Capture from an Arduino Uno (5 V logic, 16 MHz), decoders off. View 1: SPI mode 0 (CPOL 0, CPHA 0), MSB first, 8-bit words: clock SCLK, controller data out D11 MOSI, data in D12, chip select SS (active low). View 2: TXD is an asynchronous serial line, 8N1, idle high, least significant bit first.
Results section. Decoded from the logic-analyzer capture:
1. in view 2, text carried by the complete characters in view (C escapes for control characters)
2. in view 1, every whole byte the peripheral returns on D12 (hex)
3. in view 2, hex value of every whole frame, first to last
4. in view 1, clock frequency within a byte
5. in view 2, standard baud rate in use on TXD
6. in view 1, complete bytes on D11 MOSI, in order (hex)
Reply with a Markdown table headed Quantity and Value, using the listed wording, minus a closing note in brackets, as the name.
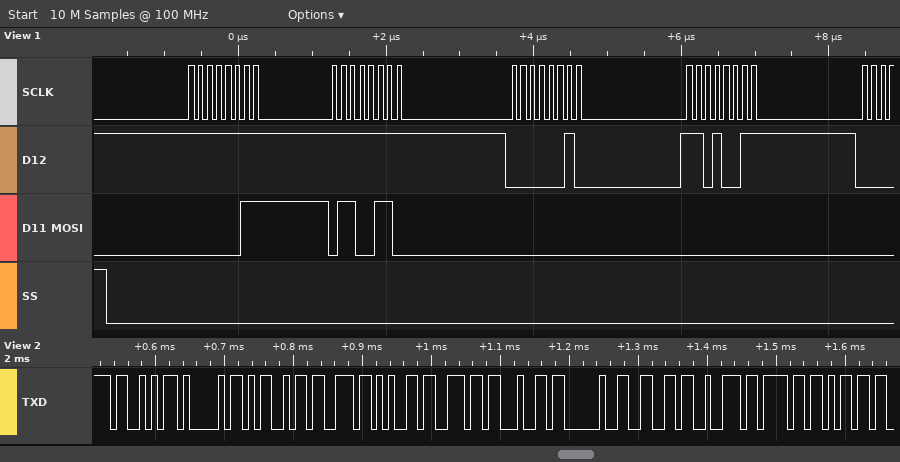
| Quantity | Value |
|---|---|
| in view 2, text carried by the complete characters in view | "SAMsend from" |
| in view 1, every whole byte the peripheral returns on D12 | FF FF 02 D3 |
| in view 2, hex value of every whole frame, first to last | 53 41 4D 73 65 6E 64 20 66 72 6F 6D |
| in view 1, clock frequency within a byte | 8 MHz |
| in view 2, standard baud rate in use on TXD | 115200 baud |
| in view 1, complete bytes on D11 MOSI, in order | 03 66 00 00 |
